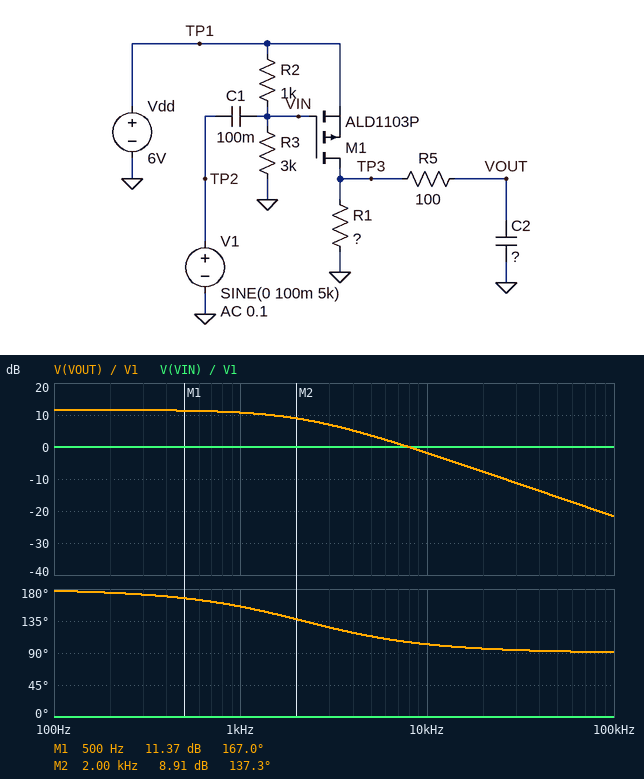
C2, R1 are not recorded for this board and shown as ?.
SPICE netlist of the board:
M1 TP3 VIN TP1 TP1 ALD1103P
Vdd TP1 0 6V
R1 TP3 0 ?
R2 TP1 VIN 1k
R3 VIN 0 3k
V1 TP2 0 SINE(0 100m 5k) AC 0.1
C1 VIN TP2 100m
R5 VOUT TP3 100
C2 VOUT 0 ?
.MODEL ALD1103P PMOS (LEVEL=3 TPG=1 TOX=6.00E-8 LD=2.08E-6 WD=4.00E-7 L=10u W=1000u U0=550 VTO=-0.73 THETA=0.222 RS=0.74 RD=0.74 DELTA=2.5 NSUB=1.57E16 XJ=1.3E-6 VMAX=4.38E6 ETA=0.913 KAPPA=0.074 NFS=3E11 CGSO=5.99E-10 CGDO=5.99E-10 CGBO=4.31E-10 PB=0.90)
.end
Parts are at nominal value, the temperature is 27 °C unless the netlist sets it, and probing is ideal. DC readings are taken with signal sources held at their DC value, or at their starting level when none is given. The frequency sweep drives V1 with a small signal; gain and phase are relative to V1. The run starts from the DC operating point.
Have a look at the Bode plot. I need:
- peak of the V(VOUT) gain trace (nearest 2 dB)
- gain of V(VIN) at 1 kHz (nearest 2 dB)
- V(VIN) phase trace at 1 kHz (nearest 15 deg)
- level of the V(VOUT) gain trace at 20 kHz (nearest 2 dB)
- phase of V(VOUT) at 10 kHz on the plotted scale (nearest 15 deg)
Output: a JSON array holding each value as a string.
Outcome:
["12 dB", "0 dB", "0 deg", "-8 dB", "105 deg"]
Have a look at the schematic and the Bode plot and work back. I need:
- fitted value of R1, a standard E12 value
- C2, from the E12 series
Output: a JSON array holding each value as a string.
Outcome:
["1.5 kΩ", "47 nF"]
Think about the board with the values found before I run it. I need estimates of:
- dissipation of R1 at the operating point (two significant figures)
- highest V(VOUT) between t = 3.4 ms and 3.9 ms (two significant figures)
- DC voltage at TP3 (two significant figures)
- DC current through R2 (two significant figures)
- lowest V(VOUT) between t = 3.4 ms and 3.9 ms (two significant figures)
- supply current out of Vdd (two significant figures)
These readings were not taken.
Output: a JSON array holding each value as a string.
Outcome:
["2.1 mW", "1.9 V", "1.8 V", "1.5 mA", "1.6 V", "2.7 mA"]
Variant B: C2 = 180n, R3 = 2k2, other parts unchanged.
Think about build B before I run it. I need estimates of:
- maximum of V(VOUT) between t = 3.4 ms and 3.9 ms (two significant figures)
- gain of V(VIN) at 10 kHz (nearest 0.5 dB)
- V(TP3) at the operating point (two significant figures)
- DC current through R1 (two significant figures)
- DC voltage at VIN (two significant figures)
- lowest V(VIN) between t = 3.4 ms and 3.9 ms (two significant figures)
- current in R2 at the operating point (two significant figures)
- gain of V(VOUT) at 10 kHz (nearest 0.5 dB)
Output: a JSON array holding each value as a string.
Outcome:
["3.5 V", "0 dB", "3.4 V", "2.3 mA", "4.1 V", "4.0 V", "1.9 mA", "-11.0 dB"]
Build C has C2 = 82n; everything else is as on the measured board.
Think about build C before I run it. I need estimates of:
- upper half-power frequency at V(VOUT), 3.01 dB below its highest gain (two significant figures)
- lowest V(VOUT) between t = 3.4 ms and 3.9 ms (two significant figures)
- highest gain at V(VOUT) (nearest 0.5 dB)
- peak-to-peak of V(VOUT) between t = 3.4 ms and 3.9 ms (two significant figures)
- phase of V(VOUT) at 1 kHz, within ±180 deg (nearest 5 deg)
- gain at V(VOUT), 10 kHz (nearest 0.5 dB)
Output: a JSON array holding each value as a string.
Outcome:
["1.2 kHz", "1.7 V", "11.5 dB", "180 mV", "140 deg", "-6.5 dB"]
